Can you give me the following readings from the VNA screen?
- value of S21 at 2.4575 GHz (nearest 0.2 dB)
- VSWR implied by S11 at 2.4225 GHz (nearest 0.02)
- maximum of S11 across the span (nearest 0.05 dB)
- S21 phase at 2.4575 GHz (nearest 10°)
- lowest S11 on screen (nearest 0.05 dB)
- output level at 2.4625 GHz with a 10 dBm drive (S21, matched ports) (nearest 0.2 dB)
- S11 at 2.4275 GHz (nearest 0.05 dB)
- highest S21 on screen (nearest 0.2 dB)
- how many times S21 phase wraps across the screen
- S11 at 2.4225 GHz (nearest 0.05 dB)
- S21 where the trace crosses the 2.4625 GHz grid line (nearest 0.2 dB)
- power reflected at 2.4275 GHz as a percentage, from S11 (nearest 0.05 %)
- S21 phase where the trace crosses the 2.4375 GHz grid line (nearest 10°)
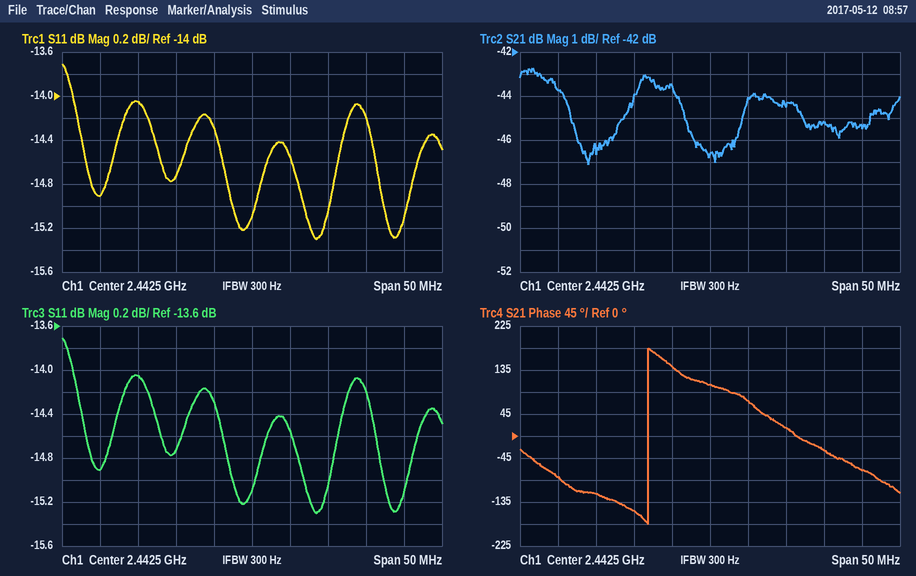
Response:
-45.2 dB
1.44
-13.70 dB
-30°
-15.30 dB
-35.4 dBm
-14.05 dB
-42.8 dB
1
-14.90 dB
-45.4 dB
3.95 %
140°
